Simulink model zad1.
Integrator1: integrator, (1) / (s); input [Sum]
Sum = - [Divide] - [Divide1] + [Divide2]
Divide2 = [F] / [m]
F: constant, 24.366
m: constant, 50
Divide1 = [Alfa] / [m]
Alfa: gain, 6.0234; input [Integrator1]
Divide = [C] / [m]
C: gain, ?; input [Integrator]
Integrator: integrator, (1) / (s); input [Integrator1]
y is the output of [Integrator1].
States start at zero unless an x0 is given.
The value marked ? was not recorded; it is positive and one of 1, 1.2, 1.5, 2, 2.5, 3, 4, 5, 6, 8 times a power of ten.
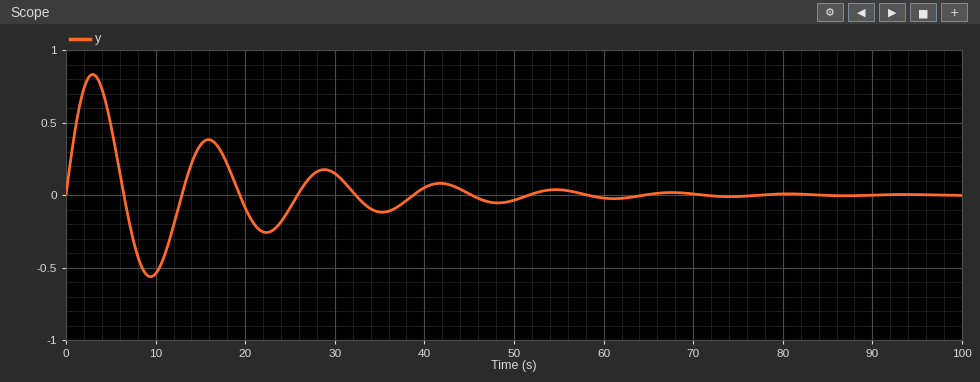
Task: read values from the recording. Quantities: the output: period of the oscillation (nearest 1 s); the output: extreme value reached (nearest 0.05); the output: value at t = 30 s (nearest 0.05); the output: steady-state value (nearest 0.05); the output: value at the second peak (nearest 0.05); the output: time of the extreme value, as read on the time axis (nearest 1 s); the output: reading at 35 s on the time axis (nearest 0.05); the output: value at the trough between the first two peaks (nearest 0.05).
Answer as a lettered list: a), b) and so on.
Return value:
a) 13 s
b) 0.85
c) 0.15
d) 0.00
e) 0.40
f) 3 s
g) -0.10
h) -0.55
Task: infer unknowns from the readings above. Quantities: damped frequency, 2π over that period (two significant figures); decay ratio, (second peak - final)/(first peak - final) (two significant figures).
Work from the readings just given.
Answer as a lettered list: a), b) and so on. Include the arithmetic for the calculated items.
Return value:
a) 2π / 13 = 0.48 rad/s
b) (0.4 - 0) / (0.85 - 0) = 0.47
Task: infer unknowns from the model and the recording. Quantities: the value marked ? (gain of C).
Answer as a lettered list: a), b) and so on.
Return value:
a) 12
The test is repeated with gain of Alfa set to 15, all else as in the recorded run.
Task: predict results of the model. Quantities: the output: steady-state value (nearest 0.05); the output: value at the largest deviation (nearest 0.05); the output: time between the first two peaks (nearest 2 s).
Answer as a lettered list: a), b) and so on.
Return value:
a) 0.00
b) 0.65
c) 14 s
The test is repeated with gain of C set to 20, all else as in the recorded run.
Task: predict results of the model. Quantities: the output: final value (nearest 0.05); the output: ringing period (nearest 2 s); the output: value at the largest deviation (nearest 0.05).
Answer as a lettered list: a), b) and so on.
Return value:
a) 0.00
b) 10 s
c) 0.65
